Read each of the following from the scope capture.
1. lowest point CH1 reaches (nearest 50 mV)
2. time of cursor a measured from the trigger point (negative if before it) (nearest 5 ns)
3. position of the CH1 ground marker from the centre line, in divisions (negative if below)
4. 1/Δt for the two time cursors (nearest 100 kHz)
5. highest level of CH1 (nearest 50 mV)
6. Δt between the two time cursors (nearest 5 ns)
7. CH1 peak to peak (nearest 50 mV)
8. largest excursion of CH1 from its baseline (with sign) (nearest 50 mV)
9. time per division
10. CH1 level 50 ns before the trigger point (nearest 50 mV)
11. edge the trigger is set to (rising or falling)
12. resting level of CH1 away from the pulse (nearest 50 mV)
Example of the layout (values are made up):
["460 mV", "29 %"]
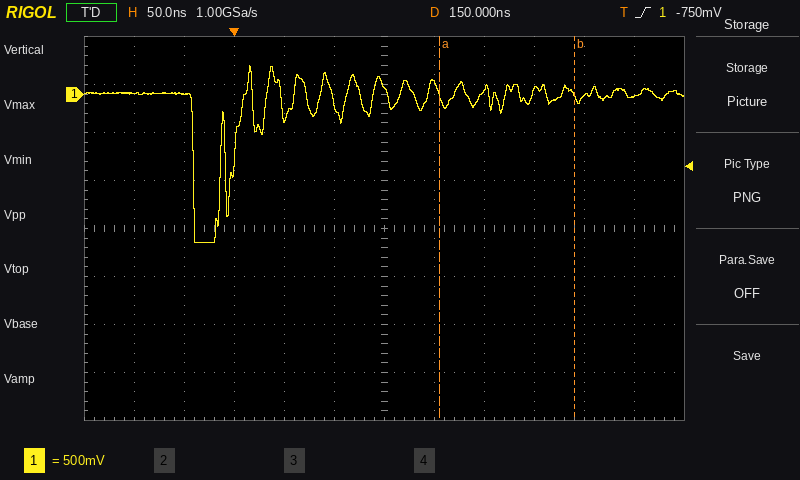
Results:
["-1.55 V", "+205 ns", "+2.8 div", "7.4 MHz", "300 mV", "135 ns", "1.85 V", "-1.55 V", "50 ns", "0 mV", "rising", "0 mV"]
